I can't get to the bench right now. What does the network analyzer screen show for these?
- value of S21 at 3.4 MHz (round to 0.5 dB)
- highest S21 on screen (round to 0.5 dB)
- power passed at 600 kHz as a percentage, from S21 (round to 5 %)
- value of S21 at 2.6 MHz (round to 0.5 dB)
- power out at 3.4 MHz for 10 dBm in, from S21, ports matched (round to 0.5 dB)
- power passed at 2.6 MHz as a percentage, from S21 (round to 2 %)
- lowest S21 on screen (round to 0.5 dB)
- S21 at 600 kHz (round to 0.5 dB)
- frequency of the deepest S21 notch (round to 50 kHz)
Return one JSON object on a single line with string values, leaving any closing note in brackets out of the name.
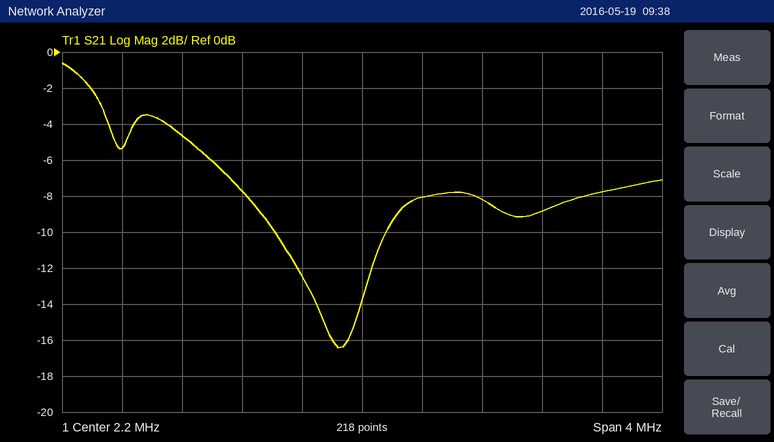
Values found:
{"value of S21 at 3.4 MHz": "-9.0 dB", "highest S21 on screen": "-0.5 dB", "power passed at 600 kHz as a percentage, from S21": "30 %", "value of S21 at 2.6 MHz": "-8.0 dB", "power out at 3.4 MHz for 10 dBm in, from S21, ports matched": "1.0 dBm", "power passed at 2.6 MHz as a percentage, from S21": "16 %", "lowest S21 on screen": "-16.5 dB", "S21 at 600 kHz": "-5.5 dB", "frequency of the deepest S21 notch": "2.05 MHz"}
